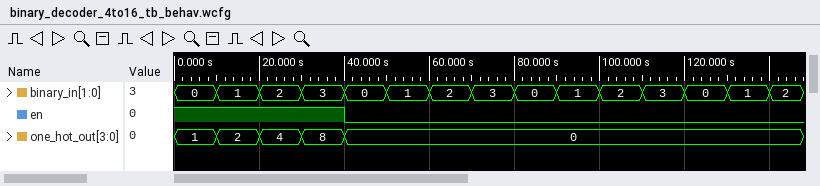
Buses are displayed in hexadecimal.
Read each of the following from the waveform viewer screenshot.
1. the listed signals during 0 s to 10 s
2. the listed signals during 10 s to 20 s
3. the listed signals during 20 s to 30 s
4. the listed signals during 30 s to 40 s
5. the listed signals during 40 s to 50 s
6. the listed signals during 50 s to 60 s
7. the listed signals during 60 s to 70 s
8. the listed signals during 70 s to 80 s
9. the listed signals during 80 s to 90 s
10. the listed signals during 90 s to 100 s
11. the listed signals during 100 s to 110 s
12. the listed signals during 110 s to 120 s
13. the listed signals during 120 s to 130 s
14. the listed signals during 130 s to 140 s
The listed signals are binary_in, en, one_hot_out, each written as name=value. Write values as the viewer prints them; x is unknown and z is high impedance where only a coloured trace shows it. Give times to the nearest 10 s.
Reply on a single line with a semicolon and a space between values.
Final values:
binary_in=0, en=1, one_hot_out=1; binary_in=1, en=1, one_hot_out=2; binary_in=2, en=1, one_hot_out=4; binary_in=3, en=1, one_hot_out=8; binary_in=0, en=0, one_hot_out=0; binary_in=1, en=0, one_hot_out=0; binary_in=2, en=0, one_hot_out=0; binary_in=3, en=0, one_hot_out=0; binary_in=0, en=0, one_hot_out=0; binary_in=1, en=0, one_hot_out=0; binary_in=2, en=0, one_hot_out=0; binary_in=3, en=0, one_hot_out=0; binary_in=0, en=0, one_hot_out=0; binary_in=1, en=0, one_hot_out=0
